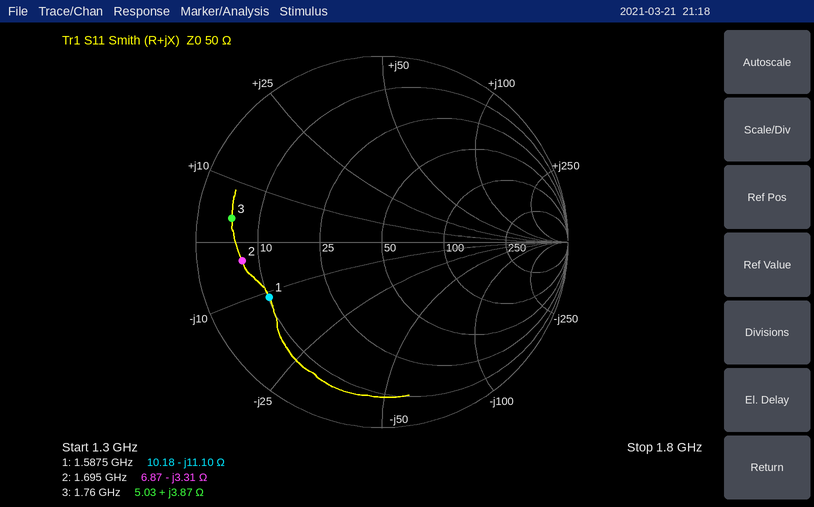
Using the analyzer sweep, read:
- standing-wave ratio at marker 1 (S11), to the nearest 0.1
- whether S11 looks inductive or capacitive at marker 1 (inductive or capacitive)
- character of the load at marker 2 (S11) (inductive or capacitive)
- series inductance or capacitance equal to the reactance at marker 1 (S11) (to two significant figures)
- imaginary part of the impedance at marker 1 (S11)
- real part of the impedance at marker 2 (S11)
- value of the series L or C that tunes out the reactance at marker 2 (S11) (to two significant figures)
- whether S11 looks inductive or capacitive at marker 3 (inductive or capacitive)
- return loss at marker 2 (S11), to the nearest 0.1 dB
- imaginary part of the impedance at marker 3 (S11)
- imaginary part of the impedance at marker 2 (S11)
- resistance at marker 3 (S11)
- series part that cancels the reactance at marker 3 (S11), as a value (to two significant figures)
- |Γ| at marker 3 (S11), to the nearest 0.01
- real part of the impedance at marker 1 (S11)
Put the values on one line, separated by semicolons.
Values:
5.2; capacitive; capacitive; 9.0 pF; -11.10 Ω; 6.87 Ω; 310 pH; inductive; 2.4 dB; +3.87 Ω; -3.31 Ω; 5.03 Ω; 23 pF; 0.82; 10.18 Ω
